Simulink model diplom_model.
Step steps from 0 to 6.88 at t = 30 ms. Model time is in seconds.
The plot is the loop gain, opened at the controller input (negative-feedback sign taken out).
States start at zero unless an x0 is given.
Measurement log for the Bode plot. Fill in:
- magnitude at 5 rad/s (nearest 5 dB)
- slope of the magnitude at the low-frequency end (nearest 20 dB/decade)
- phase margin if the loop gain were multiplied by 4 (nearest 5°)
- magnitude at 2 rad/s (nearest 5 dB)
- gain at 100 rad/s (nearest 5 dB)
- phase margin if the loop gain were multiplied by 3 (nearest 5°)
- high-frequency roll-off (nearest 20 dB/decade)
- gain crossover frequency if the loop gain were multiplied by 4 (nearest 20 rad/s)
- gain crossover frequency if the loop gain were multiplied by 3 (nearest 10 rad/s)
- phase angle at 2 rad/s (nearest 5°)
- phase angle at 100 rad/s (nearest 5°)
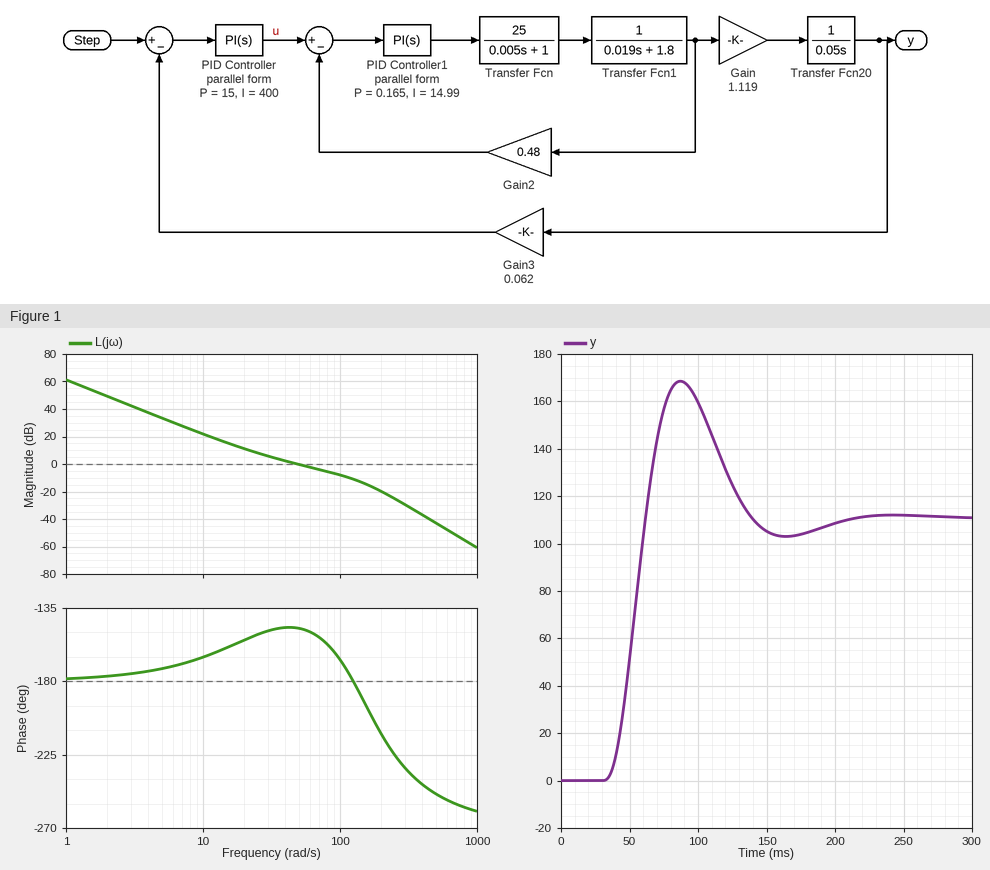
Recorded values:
35 dB
-40 dB/decade
-5°
50 dB
-10 dB
5°
-60 dB/decade
140 rad/s
110 rad/s
-175°
-165°
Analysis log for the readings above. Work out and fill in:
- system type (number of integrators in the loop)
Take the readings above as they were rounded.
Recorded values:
2
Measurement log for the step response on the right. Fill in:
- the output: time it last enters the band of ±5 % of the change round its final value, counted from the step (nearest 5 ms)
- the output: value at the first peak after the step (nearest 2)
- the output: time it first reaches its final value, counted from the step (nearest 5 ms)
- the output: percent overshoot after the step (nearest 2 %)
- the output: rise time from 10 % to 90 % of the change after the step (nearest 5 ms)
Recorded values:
155 ms
168
30 ms
52 %
20 ms
